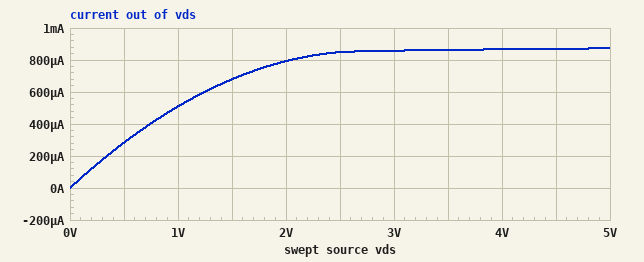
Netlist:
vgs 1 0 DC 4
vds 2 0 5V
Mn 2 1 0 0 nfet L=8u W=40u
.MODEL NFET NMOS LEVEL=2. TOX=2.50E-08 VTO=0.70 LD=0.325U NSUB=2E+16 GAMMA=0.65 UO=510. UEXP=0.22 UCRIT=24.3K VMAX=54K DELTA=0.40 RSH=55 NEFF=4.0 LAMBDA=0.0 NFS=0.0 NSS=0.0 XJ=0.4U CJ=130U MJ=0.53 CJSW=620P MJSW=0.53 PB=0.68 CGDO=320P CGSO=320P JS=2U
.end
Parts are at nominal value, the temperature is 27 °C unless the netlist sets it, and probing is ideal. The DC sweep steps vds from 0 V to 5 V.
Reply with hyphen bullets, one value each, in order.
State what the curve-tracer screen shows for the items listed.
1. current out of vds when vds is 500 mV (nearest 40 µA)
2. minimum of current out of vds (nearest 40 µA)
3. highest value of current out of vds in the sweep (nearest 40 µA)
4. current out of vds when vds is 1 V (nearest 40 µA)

- 280 µA
- 0 A
- 880 µA
- 520 µA
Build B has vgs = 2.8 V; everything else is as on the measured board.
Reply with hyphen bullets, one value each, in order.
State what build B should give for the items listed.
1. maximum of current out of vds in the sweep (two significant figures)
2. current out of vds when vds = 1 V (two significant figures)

- 390 µA
- 320 µA
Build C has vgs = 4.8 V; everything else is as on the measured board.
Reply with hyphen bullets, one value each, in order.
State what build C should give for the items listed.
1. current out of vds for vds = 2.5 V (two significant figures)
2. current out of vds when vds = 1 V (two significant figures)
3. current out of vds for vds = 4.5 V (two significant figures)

- 1.2 mA
- 620 µA
- 1.3 mA
